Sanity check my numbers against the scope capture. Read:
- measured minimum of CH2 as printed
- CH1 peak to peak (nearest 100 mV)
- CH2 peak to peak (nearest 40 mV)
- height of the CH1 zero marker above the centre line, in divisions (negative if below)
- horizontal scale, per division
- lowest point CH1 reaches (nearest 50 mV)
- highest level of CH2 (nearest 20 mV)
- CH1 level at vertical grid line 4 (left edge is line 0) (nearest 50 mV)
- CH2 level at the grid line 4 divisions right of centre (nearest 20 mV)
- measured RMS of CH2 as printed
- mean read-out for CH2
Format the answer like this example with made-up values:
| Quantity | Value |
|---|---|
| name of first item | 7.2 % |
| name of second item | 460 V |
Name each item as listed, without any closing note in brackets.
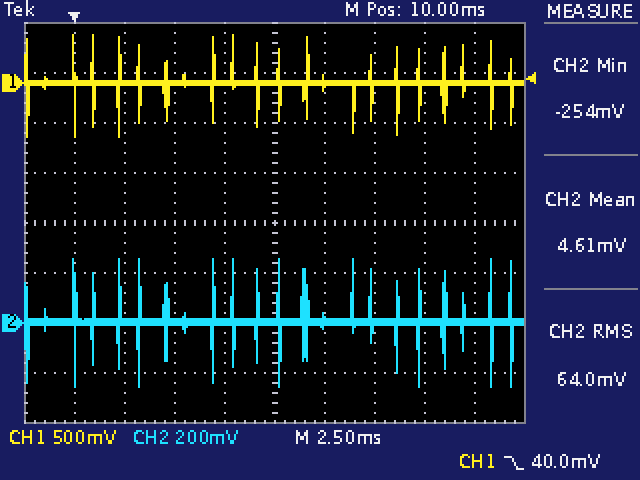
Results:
| Quantity | Value |
|---|---|
| measured minimum of CH2 as printed | -254 mV |
| CH1 peak to peak | 1.00 V |
| CH2 peak to peak | 520 mV |
| height of the CH1 zero marker above the centre line, in divisions | +2.8 div |
| horizontal scale, per division | 2.5 ms |
| lowest point CH1 reaches | -550 mV |
| highest level of CH2 | 260 mV |
| CH1 level at vertical grid line 4 (left edge is line 0) | 0 mV |
| CH2 level at the grid line 4 divisions right of centre | 0 mV |
| measured RMS of CH2 as printed | 64.0 mV |
| mean read-out for CH2 | 4.61 mV |
